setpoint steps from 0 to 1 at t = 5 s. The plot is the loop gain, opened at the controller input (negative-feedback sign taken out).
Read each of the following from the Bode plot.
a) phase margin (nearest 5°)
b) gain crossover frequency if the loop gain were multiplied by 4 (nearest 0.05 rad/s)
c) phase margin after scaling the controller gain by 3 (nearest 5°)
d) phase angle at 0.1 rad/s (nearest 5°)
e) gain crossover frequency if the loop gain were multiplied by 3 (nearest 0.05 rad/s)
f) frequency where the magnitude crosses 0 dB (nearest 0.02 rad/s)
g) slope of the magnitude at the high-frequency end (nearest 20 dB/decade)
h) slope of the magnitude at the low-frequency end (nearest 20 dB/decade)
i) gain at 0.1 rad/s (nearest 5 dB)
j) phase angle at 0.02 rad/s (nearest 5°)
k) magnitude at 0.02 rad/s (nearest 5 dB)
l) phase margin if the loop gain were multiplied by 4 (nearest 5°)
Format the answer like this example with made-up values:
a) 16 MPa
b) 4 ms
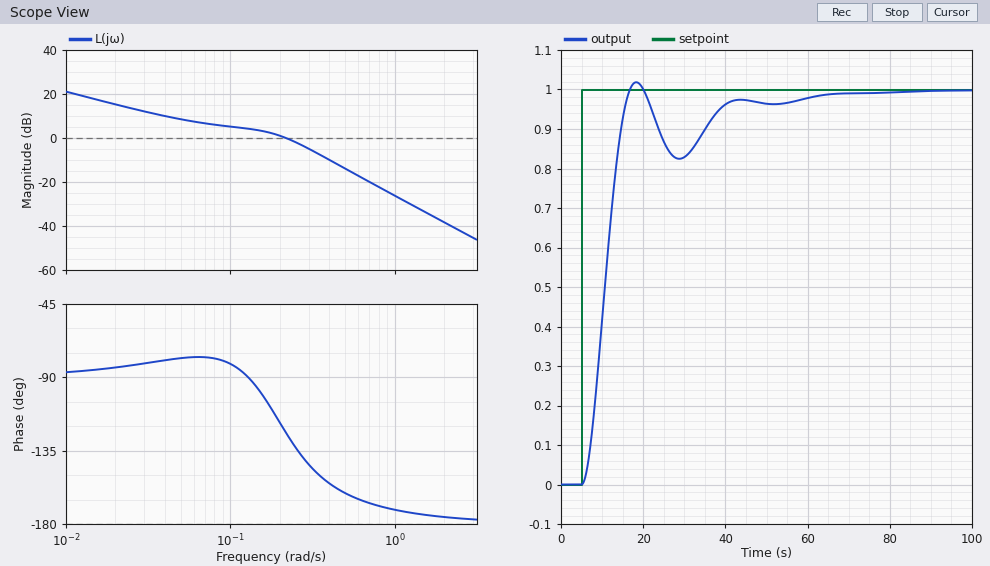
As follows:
a) 55°
b) 0.45 rad/s
c) 25°
d) -80°
e) 0.40 rad/s
f) 0.22 rad/s
g) -40 dB/decade
h) -20 dB/decade
i) 5 dB
j) -85°
k) 15 dB
l) 20°
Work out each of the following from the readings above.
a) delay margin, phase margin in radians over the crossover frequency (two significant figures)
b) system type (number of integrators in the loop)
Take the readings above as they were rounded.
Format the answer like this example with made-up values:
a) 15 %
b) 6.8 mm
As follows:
a) 4.4 s
b) 1
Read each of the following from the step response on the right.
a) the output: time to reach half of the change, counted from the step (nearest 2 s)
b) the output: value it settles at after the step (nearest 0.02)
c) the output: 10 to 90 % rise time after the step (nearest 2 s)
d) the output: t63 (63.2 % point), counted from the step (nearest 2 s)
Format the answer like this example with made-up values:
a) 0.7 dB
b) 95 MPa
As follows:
a) 6 s
b) 1.00
c) 8 s
d) 6 s
